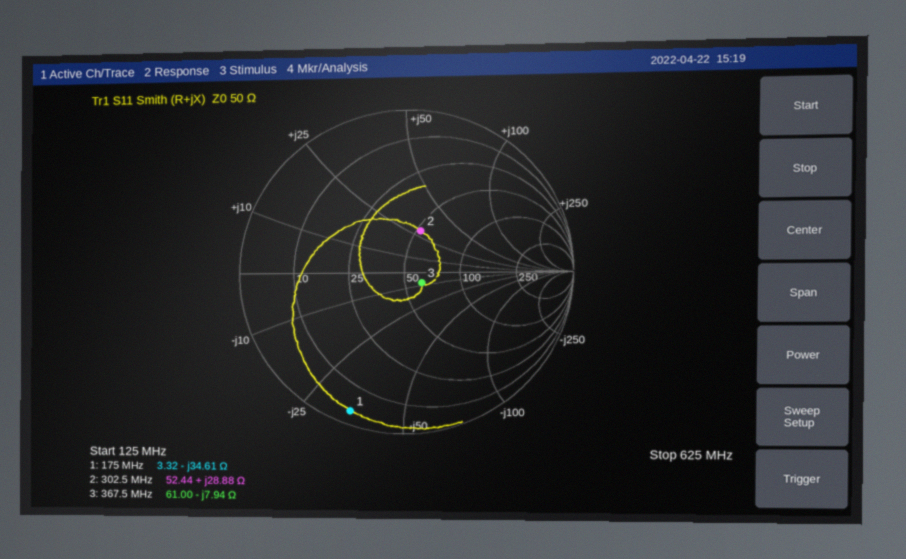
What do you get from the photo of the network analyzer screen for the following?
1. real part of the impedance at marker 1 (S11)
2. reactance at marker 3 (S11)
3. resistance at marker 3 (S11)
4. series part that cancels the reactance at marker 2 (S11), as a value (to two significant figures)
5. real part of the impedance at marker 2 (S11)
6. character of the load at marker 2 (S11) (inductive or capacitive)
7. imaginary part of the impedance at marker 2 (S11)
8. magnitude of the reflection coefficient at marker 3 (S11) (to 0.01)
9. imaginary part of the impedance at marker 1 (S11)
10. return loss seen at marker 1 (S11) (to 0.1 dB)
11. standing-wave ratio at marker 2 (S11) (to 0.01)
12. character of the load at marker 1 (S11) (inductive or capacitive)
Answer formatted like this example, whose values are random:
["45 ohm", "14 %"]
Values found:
["3.32 Ω", "-7.94 Ω", "61.00 Ω", "18 pF", "52.44 Ω", "inductive", "+28.88 Ω", "0.12", "-34.61 Ω", "0.8 dB", "1.75", "capacitive"]
